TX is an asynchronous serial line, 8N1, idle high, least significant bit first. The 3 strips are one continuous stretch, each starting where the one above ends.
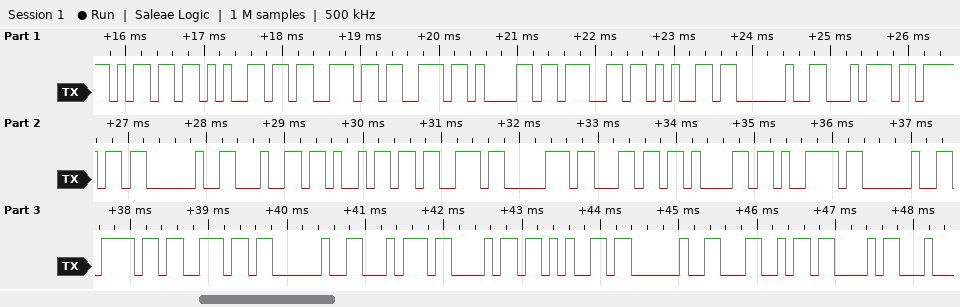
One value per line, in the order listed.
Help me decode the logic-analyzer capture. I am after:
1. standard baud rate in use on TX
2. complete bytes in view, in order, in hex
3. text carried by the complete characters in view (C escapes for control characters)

9600 baud
6D 65 73 73 61 67 65 20 74 6F 20 64 69 73 70 6C 61 79 20 6F 6E 20 74 68 65 20 4C 43
"message to display on the LC"
